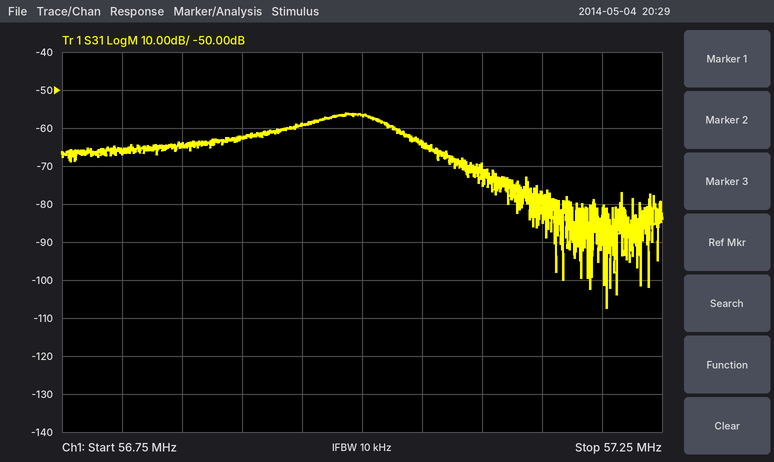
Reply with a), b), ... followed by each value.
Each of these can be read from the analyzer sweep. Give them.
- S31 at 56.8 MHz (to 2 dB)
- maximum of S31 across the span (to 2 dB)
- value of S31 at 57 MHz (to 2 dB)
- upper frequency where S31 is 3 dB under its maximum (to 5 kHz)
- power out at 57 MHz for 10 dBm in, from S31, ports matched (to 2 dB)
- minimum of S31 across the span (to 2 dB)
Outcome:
a) -66 dB
b) -56 dB
c) -56 dB
d) 57.020 MHz
e) -46 dBm
f) -108 dB
